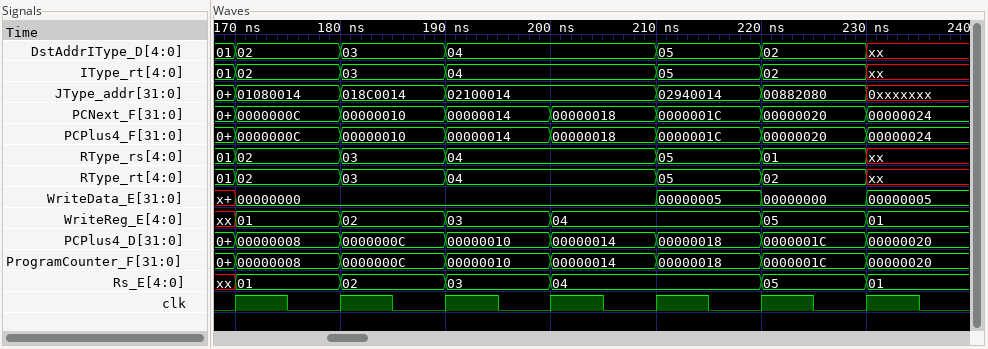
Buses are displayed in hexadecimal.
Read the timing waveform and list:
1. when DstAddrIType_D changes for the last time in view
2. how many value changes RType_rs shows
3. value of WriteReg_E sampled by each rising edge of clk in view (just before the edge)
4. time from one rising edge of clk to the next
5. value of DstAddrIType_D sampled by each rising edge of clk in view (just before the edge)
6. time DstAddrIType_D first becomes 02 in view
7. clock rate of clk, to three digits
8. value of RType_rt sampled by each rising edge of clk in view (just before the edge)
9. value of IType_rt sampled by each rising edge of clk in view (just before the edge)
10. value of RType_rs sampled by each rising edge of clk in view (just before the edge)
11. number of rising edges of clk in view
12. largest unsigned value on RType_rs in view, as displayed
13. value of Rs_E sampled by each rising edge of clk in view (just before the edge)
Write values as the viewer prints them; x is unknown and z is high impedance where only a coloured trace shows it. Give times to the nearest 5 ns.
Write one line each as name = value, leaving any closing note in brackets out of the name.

when DstAddrIType_D changes for the last time in view = 230 ns
how many value changes RType_rs shows = 6
value of WriteReg_E sampled by each rising edge of clk in view = xx, 01, 02, 03, 04, 04, 05
time from one rising edge of clk to the next = 10 ns
value of DstAddrIType_D sampled by each rising edge of clk in view = 01, 02, 03, 04, 04, 05, 02
time DstAddrIType_D first becomes 02 in view = 170 ns
clock rate of clk, to three digits = 100 MHz
value of RType_rt sampled by each rising edge of clk in view = 01, 02, 03, 04, 04, 05, 02
value of IType_rt sampled by each rising edge of clk in view = 01, 02, 03, 04, 04, 05, 02
value of RType_rs sampled by each rising edge of clk in view = 01, 02, 03, 04, 04, 05, 01
number of rising edges of clk in view = 7
largest unsigned value on RType_rs in view, as displayed = 05
value of Rs_E sampled by each rising edge of clk in view = xx, 01, 02, 03, 04, 04, 05
